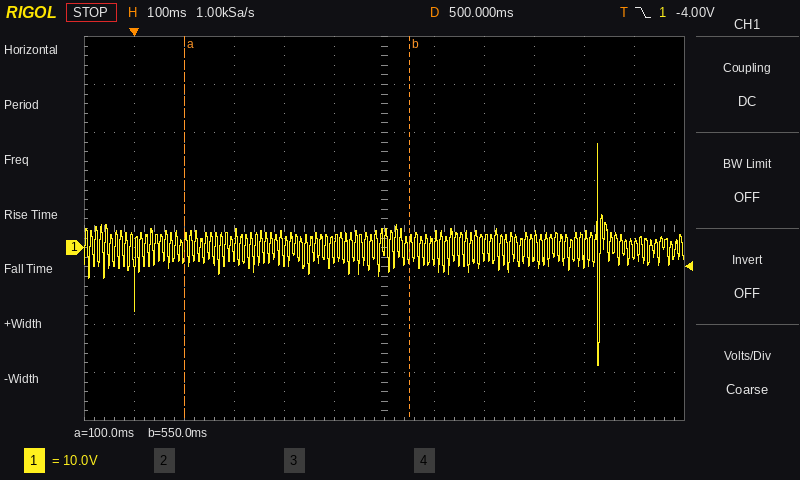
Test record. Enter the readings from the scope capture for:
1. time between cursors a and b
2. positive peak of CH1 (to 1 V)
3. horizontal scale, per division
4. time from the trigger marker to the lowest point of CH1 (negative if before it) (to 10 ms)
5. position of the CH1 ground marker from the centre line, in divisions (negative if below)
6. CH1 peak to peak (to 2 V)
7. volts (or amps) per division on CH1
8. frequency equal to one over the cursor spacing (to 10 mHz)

450 ms
22 V
100 ms
+930 ms
-0.4 div
46 V
10 V
2.22 Hz
